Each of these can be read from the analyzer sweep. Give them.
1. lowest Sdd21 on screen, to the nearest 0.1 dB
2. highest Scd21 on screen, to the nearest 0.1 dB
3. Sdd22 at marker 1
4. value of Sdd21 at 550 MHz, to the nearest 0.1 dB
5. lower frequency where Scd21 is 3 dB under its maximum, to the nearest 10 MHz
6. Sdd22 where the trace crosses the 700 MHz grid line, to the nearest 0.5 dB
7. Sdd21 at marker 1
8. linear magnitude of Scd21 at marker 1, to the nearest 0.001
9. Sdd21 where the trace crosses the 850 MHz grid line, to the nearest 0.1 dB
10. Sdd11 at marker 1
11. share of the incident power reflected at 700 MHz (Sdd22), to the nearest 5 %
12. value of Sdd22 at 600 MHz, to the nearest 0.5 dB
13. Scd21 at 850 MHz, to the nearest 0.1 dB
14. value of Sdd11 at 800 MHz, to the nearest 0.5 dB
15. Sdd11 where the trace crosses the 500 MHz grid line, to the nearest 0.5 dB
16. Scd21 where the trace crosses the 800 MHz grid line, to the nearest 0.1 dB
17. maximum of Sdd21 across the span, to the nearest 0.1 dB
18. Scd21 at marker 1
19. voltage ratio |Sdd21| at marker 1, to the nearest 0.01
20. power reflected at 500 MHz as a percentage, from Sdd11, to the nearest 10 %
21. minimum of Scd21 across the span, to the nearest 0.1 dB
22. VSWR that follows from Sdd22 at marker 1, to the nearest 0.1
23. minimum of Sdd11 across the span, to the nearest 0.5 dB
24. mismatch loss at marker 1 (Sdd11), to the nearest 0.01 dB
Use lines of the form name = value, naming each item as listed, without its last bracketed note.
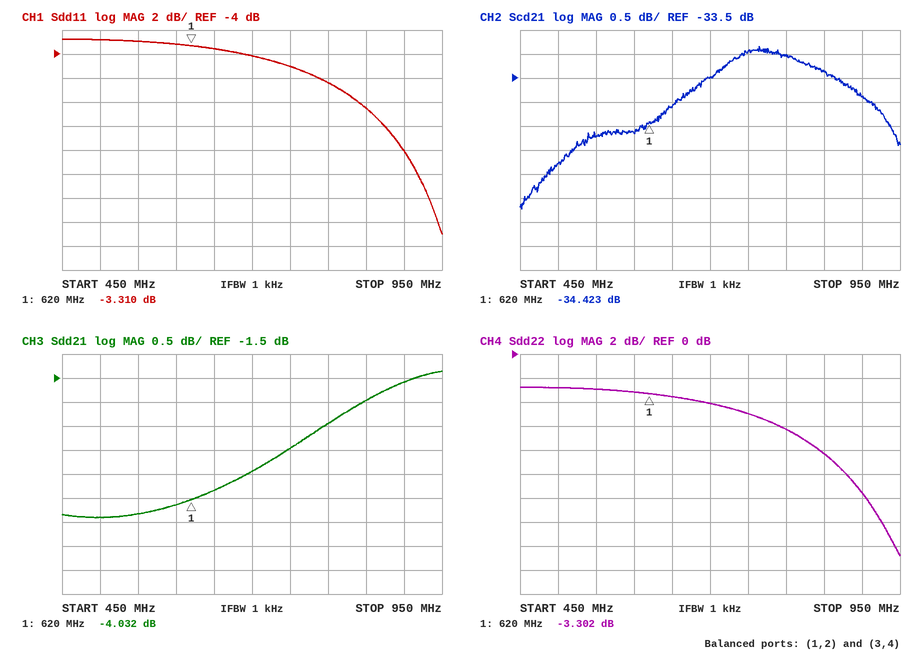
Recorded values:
lowest Sdd21 on screen, to the nearest 0.1 dB = -4.4 dB
highest Scd21 on screen, to the nearest 0.1 dB = -32.8 dB
Sdd22 at marker 1 = -3.302 dB
value of Sdd21 at 550 MHz, to the nearest 0.1 dB = -4.3 dB
lower frequency where Scd21 is 3 dB under its maximum, to the nearest 10 MHz = 470 MHz
Sdd22 where the trace crosses the 700 MHz grid line, to the nearest 0.5 dB = -4.0 dB
Sdd21 at marker 1 = -4.032 dB
linear magnitude of Scd21 at marker 1, to the nearest 0.001 = 0.019
Sdd21 where the trace crosses the 850 MHz grid line, to the nearest 0.1 dB = -2.0 dB
Sdd11 at marker 1 = -3.310 dB
share of the incident power reflected at 700 MHz (Sdd22), to the nearest 5 % = 40 %
value of Sdd22 at 600 MHz, to the nearest 0.5 dB = -3.0 dB
Scd21 at 850 MHz, to the nearest 0.1 dB = -33.4 dB
value of Sdd11 at 800 MHz, to the nearest 0.5 dB = -6.5 dB
Sdd11 where the trace crosses the 500 MHz grid line, to the nearest 0.5 dB = -3.0 dB
Scd21 where the trace crosses the 800 MHz grid line, to the nearest 0.1 dB = -33.0 dB
maximum of Sdd21 across the span, to the nearest 0.1 dB = -1.4 dB
Scd21 at marker 1 = -34.423 dB
voltage ratio |Sdd21| at marker 1, to the nearest 0.01 = 0.63
power reflected at 500 MHz as a percentage, from Sdd11, to the nearest 10 % = 50 %
minimum of Scd21 across the span, to the nearest 0.1 dB = -36.2 dB
VSWR that follows from Sdd22 at marker 1, to the nearest 0.1 = 5.3
minimum of Sdd11 across the span, to the nearest 0.5 dB = -19.0 dB
mismatch loss at marker 1 (Sdd11), to the nearest 0.01 dB = 2.73 dB
